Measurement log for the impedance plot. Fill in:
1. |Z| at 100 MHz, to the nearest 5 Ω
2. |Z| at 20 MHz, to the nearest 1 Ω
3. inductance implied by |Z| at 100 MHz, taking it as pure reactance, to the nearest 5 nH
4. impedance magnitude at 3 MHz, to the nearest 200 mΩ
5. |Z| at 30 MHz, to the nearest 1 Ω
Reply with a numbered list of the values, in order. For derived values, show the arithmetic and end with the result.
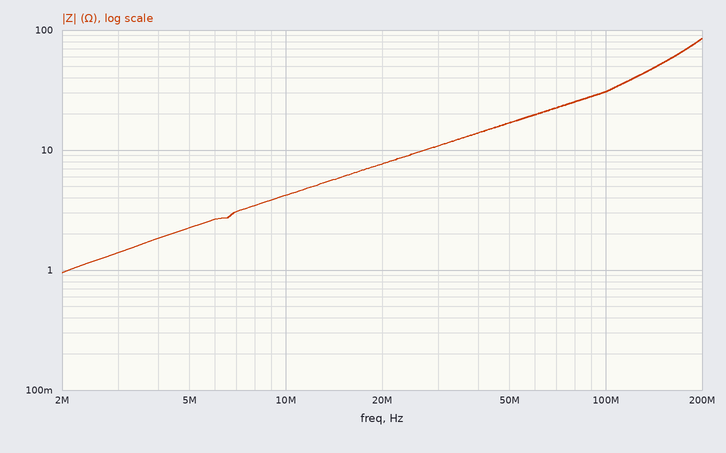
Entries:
1. 30 Ω
2. 8 Ω
3. L = 30 Ω/(2π × 100 MHz) ≈ 47.7 nH, so 50 nH to the nearest 5 nH
4. 1.4 Ω
5. 11 Ω
